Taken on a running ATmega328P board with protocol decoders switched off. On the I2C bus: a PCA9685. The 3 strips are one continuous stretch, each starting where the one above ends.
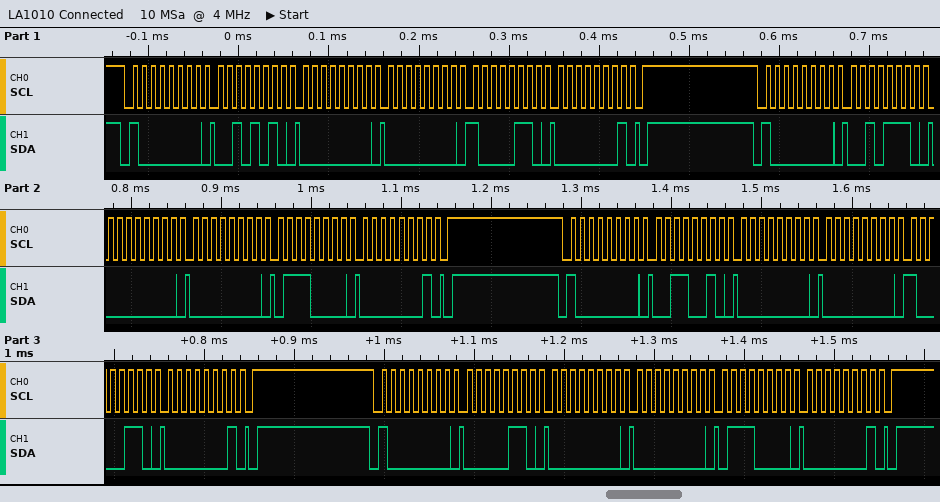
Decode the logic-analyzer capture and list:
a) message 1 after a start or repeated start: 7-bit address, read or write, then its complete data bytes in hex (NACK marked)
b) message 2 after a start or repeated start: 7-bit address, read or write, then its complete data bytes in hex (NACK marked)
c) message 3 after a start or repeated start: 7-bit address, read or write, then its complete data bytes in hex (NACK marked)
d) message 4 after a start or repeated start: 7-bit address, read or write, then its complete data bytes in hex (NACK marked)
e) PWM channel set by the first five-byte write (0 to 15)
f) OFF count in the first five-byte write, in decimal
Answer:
0x40 write: 2A 00 00 86 01
0x40 write: 2E 00 00 70 01
0x40 write: 32 00 00 86 01
0x40 write: 06 00 00 70 01
9
390
